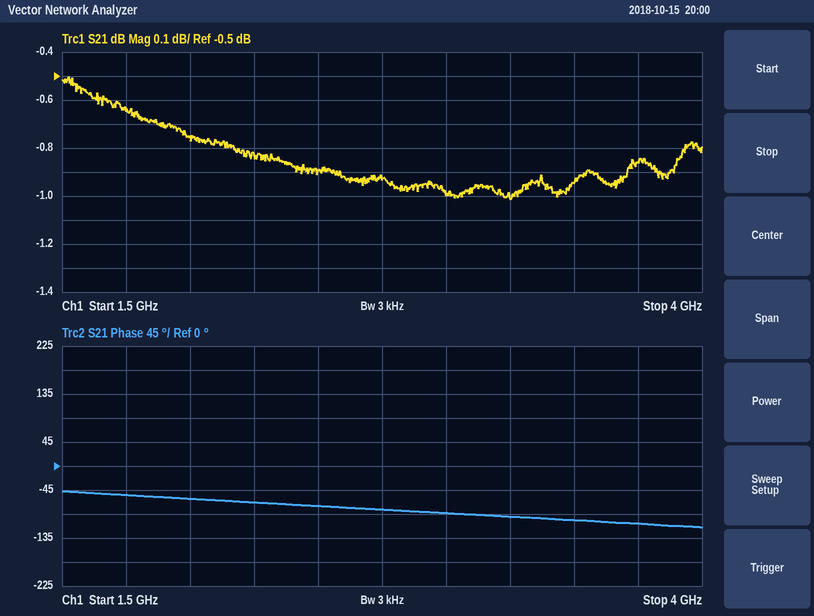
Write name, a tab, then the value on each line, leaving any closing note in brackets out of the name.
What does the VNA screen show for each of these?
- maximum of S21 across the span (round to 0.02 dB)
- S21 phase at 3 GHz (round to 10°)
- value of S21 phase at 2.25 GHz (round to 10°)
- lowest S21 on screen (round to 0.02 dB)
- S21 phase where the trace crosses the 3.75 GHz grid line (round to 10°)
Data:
maximum of S21 across the span	-0.50 dB
S21 phase at 3 GHz	-90°
value of S21 phase at 2.25 GHz	-70°
lowest S21 on screen	-1.02 dB
S21 phase where the trace crosses the 3.75 GHz grid line	-110°
